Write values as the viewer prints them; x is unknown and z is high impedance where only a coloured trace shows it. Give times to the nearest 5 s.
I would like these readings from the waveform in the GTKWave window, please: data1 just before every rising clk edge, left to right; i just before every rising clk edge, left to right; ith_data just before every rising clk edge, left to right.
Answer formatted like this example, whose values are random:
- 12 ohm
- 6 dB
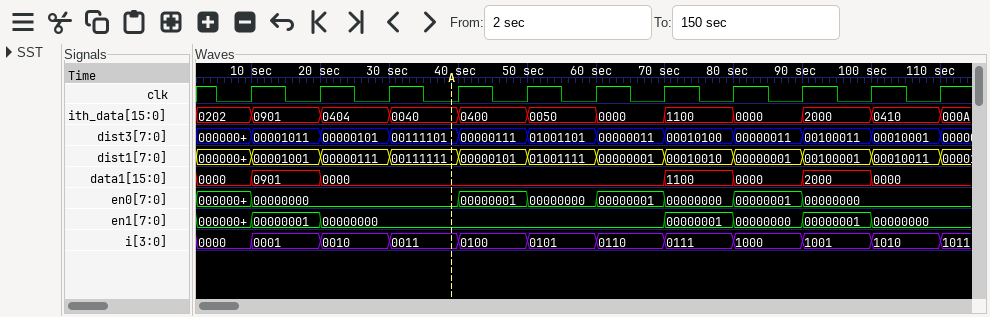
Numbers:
- 0000, 0901, 0000, 0000, 0000, 0000, 0000, 1100, 0000, 2000, 0000
- 0000, 0001, 0010, 0011, 0100, 0101, 0110, 0111, 1000, 1001, 1010
- 0202, 0901, 0404, 0040, 0400, 0050, 0000, 1100, 0000, 2000, 0410
